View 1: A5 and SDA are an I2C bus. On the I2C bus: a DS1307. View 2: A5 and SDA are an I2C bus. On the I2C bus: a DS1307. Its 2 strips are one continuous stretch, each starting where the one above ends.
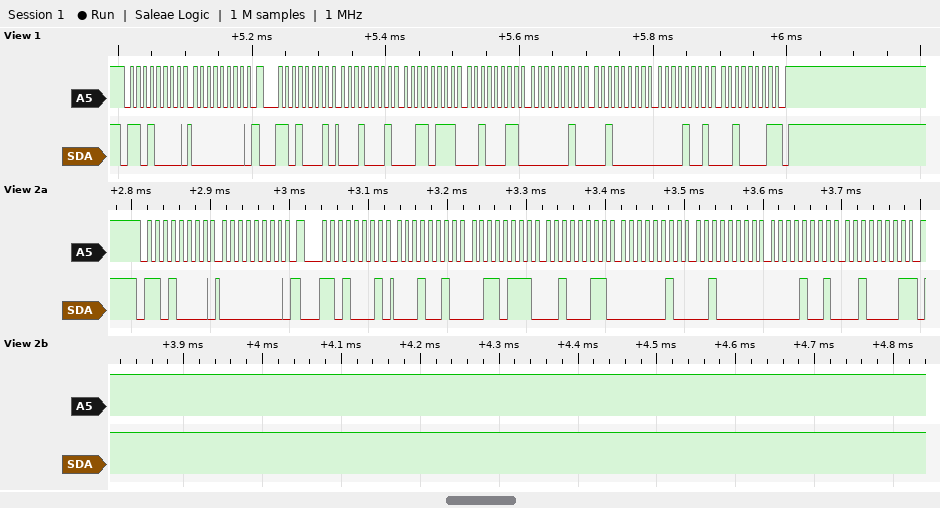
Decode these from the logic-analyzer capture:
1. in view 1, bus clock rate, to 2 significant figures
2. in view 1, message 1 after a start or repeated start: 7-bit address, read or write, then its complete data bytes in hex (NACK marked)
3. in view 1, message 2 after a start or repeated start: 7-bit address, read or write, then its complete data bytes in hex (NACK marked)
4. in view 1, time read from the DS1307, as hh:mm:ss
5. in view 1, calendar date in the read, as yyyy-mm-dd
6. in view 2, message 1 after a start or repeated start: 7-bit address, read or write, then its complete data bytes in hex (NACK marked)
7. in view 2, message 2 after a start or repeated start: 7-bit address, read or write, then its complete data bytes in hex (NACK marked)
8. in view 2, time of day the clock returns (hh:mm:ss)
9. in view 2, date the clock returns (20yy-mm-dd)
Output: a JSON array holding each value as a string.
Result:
["100 kHz", "0x68 write: 00", "0x68 read: 11 37 23 02 20 09 21 NACK", "23:37:11", "2021-09-20", "0x68 write: 00", "0x68 read: 12 37 23 02 20 09 21 NACK", "23:37:12", "2021-09-20"]
